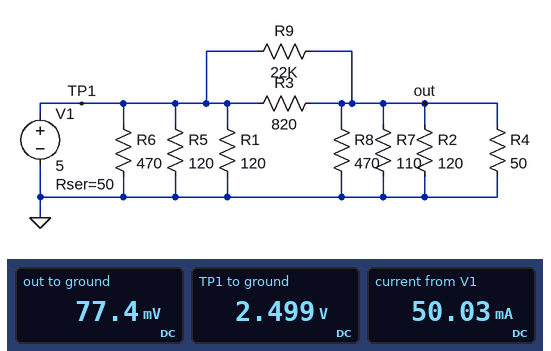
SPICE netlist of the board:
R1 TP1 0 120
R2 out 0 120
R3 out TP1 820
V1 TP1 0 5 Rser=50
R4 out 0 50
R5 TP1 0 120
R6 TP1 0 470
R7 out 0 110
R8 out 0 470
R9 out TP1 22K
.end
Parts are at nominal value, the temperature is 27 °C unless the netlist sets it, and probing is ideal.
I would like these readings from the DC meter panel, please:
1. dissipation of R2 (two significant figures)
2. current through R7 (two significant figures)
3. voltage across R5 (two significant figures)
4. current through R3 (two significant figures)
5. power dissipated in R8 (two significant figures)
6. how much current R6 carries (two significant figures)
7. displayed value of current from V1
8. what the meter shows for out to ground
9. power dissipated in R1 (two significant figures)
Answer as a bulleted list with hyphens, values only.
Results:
- 50 µW
- 700 µA
- 2.5 V
- 3.0 mA
- 13 µW
- 5.3 mA
- 50.03 mA
- 77.4 mV
- 52 mW
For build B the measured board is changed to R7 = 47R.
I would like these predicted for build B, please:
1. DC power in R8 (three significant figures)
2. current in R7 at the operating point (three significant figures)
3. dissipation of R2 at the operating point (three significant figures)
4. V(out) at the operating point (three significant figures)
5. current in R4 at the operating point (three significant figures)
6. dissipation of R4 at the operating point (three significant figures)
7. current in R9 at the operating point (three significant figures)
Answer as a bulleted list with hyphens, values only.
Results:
- 7.56 µW
- 1.27 mA
- 29.6 µW
- 59.6 mV
- 1.19 mA
- 71.1 µW
- 111 µA
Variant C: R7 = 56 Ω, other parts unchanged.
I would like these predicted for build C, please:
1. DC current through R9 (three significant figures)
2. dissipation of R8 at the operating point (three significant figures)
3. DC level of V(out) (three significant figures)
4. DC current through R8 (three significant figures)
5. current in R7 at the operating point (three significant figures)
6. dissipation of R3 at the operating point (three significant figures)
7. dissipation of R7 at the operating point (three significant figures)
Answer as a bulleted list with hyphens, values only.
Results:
- 111 µA
- 8.64 µW
- 63.7 mV
- 136 µA
- 1.14 mA
- 7.23 mW
- 72.5 µW
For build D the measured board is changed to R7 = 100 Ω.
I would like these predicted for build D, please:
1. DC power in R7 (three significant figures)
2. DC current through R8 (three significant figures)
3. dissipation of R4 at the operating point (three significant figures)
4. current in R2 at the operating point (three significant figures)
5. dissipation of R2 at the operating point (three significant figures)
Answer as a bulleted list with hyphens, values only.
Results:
- 57.4 µW
- 161 µA
- 115 µW
- 631 µA
- 47.8 µW
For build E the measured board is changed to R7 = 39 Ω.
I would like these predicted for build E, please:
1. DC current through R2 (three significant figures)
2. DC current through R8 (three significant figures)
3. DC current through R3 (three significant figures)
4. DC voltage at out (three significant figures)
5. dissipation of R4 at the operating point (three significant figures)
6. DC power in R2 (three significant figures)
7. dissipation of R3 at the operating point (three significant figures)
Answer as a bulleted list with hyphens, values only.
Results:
- 459 µA
- 117 µA
- 2.98 mA
- 55.1 mV
- 60.7 µW
- 25.3 µW
- 7.28 mW
